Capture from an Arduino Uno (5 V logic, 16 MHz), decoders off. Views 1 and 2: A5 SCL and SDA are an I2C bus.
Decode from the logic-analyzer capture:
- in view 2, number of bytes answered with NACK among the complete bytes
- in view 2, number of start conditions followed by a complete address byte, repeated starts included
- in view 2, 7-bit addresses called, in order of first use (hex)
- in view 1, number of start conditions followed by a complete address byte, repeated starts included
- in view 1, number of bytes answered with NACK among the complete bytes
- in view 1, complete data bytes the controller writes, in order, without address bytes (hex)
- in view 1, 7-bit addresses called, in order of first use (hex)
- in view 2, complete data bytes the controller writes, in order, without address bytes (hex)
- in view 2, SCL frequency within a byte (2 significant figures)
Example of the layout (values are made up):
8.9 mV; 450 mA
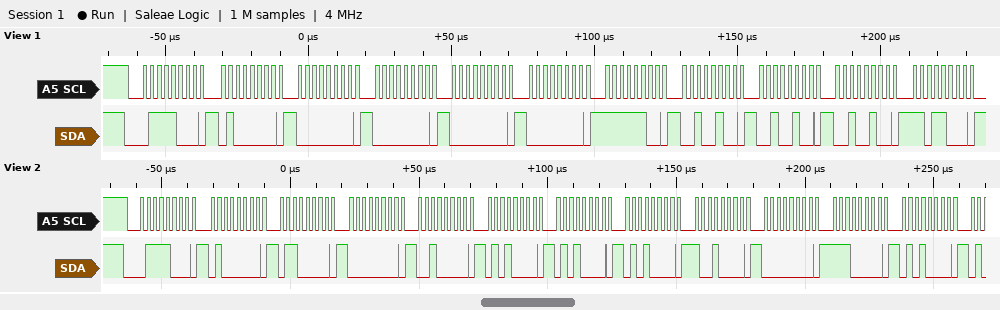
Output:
0; 1; 0x3C; 1; 0; 40 00 00 00 00 FC 24 24 24 D8; 0x3C; 40 60 00 20 50 50 50 90 00 E0 50; 400 kHz
